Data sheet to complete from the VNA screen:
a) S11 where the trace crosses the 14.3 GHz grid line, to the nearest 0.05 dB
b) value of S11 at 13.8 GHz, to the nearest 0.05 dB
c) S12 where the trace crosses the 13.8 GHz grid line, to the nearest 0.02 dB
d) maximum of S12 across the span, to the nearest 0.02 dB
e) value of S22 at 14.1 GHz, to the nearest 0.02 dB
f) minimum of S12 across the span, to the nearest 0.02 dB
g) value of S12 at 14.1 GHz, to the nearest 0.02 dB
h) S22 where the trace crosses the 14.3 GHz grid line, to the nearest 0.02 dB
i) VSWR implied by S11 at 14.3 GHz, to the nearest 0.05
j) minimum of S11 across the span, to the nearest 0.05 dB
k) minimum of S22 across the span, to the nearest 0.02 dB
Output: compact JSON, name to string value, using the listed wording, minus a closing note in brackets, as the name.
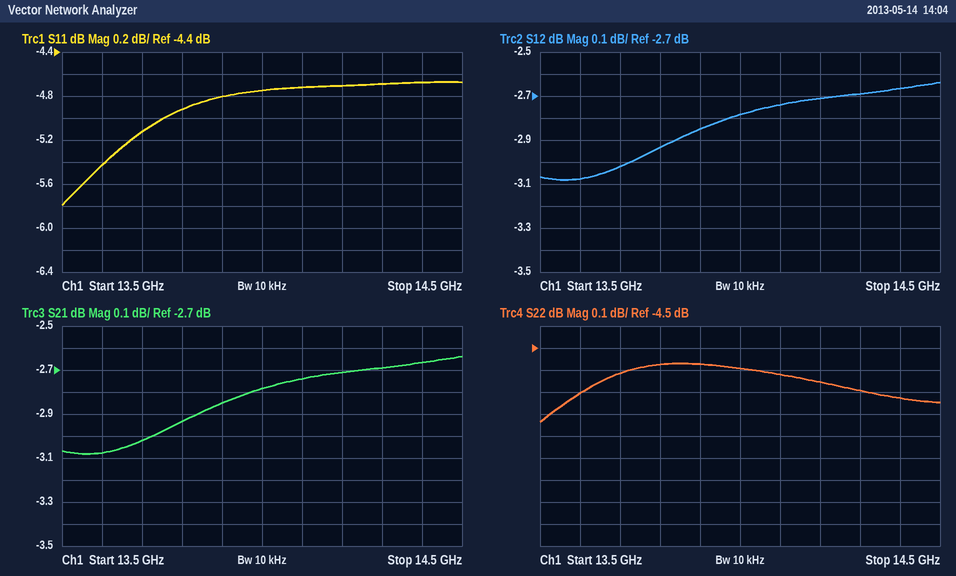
{"S11 where the trace crosses the 14.3 GHz grid line, to the nearest 0.05 dB": "-4.70 dB", "value of S11 at 13.8 GHz, to the nearest 0.05 dB": "-4.90 dB", "S12 where the trace crosses the 13.8 GHz grid line, to the nearest 0.02 dB": "-2.94 dB", "maximum of S12 across the span, to the nearest 0.02 dB": "-2.64 dB", "value of S22 at 14.1 GHz, to the nearest 0.02 dB": "-4.62 dB", "minimum of S12 across the span, to the nearest 0.02 dB": "-3.08 dB", "value of S12 at 14.1 GHz, to the nearest 0.02 dB": "-2.74 dB", "S22 where the trace crosses the 14.3 GHz grid line, to the nearest 0.02 dB": "-4.70 dB", "VSWR implied by S11 at 14.3 GHz, to the nearest 0.05": "3.80", "minimum of S11 across the span, to the nearest 0.05 dB": "-5.80 dB", "minimum of S22 across the span, to the nearest 0.02 dB": "-4.84 dB"}
